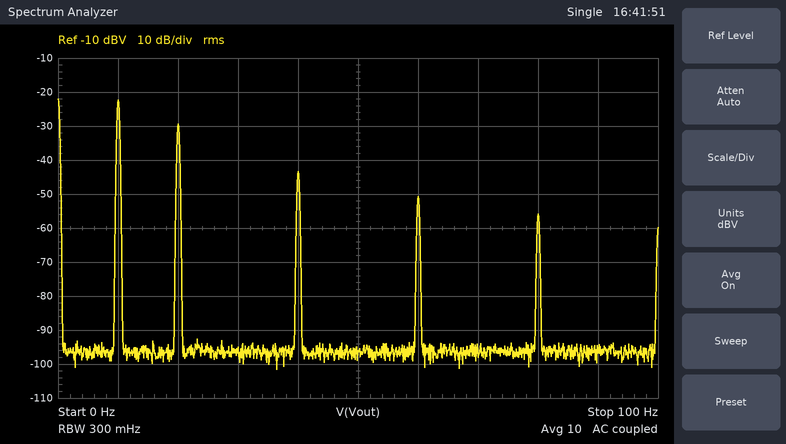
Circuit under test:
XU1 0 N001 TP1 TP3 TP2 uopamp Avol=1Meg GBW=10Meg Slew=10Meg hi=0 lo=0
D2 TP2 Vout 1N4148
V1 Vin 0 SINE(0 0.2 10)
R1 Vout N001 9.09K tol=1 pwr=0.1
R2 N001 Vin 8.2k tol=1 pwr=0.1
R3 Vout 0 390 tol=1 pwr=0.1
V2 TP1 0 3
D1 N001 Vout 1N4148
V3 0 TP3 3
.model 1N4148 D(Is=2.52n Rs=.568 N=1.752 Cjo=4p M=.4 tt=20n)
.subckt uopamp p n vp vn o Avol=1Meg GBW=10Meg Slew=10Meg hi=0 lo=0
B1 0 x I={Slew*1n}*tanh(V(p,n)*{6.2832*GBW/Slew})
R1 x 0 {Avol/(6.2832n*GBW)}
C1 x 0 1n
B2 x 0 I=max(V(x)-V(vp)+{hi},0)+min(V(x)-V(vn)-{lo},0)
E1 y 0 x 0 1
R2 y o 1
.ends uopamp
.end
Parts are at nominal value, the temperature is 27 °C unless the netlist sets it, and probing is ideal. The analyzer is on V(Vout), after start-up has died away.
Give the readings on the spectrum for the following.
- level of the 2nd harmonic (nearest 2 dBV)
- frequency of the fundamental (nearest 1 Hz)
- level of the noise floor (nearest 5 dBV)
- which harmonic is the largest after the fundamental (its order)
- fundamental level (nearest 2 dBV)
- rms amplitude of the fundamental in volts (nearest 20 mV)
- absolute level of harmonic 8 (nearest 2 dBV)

-30 dBV
10 Hz
-95 dBV
2
-22 dBV
80 mV
-56 dBV
